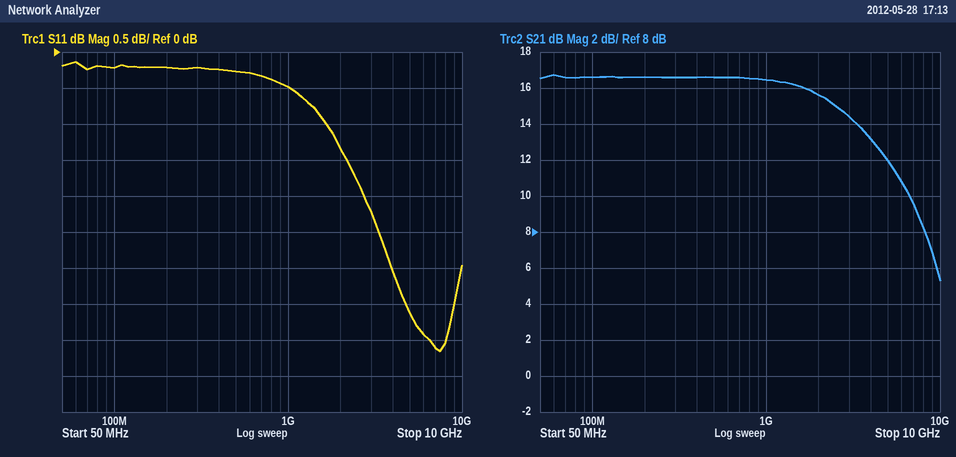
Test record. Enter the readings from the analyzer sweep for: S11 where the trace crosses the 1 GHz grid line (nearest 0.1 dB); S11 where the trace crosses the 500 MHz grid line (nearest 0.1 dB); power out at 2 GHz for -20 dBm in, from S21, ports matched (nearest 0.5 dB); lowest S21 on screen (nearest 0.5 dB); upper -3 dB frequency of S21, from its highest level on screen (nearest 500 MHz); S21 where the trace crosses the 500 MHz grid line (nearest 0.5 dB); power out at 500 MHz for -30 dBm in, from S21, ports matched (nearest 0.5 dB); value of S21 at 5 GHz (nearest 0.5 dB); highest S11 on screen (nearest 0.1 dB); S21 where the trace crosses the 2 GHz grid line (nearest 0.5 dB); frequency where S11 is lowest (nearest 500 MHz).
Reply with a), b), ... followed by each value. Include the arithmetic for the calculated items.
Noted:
a) -0.5 dB
b) -0.3 dB
c) -20 dBm + (15.5 dB) = -4.5 dBm
d) 5.5 dB
e) 3.5 GHz
f) 16.5 dB
g) -30 dBm + (16.5 dB) = -13.5 dBm
h) 12.0 dB
i) -0.1 dB
j) 15.5 dB
k) 7.5 GHz
